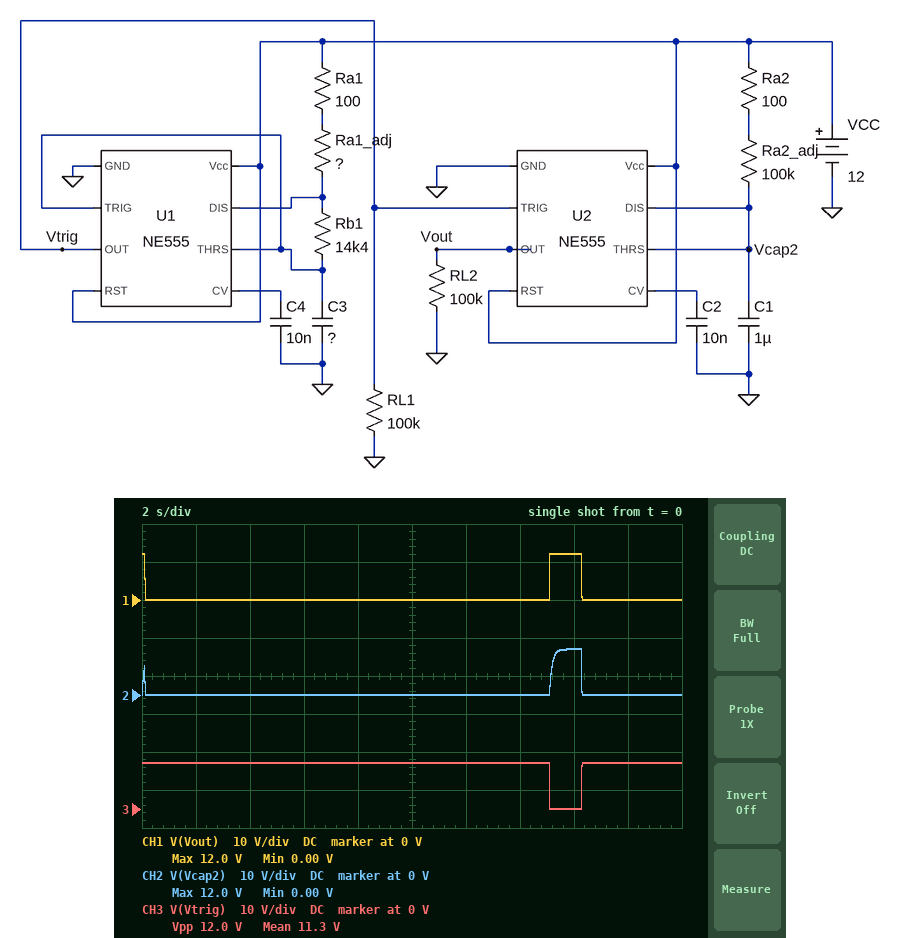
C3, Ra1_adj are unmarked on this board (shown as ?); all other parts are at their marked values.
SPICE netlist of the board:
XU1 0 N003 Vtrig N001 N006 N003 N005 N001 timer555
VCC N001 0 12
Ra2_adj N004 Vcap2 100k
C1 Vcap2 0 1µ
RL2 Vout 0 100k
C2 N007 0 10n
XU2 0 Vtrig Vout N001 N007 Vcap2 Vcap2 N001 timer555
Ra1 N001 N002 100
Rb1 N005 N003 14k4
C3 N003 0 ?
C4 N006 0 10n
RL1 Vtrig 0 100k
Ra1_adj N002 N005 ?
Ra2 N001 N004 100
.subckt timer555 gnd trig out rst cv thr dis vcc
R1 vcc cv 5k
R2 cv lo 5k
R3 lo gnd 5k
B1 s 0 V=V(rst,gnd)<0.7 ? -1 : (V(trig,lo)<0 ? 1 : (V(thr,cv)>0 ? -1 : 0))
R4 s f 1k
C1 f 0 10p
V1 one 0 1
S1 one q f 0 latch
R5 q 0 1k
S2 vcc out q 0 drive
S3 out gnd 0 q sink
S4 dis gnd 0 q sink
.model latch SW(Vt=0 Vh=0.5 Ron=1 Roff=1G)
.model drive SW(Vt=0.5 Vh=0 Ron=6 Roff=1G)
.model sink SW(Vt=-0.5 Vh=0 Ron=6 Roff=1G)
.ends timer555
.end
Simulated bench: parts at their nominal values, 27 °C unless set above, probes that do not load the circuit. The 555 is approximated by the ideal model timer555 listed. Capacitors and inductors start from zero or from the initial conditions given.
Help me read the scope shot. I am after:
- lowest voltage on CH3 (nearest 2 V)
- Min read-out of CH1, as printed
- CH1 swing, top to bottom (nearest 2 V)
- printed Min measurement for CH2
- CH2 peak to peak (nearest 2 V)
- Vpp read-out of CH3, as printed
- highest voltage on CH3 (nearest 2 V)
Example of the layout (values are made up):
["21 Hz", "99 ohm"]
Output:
["0 V", "0.00 V", "12 V", "0.00 V", "12 V", "12.0 V", "12 V"]
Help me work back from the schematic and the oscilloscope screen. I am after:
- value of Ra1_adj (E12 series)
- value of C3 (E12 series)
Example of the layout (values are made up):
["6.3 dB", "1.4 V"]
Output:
["100 kΩ", "120 µF"]
